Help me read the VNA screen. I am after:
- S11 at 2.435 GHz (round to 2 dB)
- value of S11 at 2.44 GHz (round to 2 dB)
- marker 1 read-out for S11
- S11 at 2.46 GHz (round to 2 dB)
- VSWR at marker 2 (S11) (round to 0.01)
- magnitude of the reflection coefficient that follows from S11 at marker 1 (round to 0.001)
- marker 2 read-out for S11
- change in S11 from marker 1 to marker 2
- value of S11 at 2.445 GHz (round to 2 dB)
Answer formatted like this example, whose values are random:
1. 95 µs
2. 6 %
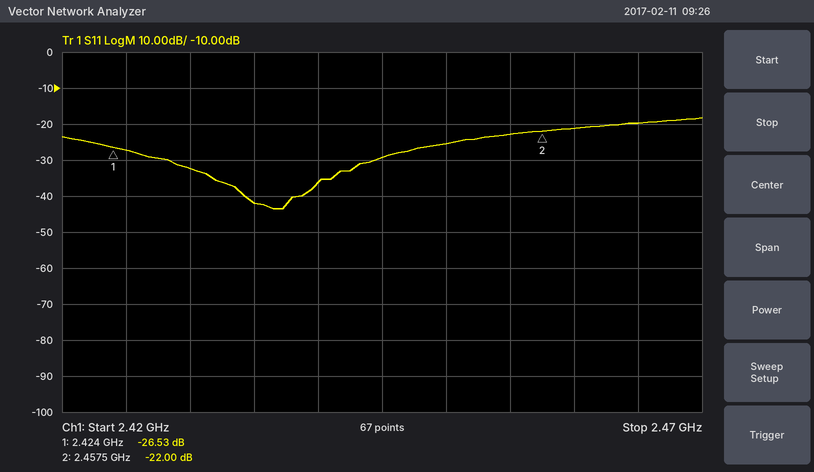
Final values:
1. -42 dB
2. -36 dB
3. -26.53 dB
4. -22 dB
5. 1.17
6. 0.047
7. -22.00 dB
8. 4.53 dB
9. -30 dB
